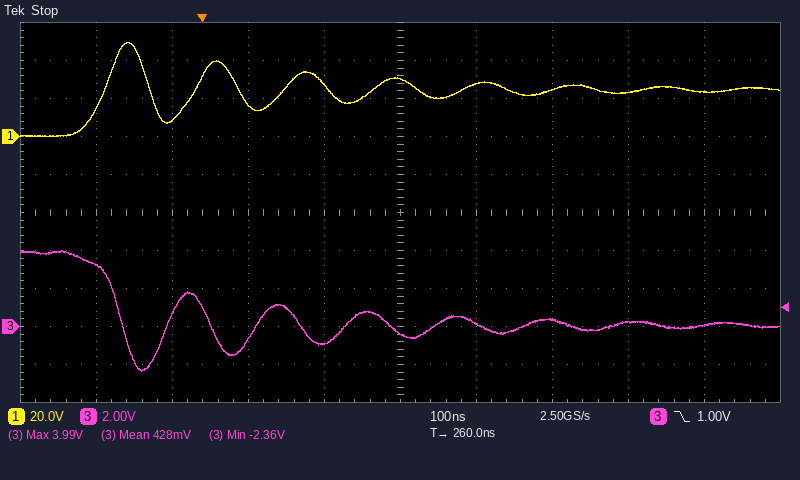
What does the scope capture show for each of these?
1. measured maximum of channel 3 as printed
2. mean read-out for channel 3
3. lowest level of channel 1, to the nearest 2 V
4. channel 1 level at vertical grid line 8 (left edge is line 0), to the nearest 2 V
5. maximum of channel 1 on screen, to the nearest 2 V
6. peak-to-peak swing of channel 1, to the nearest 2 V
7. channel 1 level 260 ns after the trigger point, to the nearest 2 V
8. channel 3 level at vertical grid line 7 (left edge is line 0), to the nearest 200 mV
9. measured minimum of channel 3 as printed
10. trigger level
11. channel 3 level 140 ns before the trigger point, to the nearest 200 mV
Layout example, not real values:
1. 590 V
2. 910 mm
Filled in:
1. 3.99 V
2. 428 mV
3. 0 V
4. 24 V
5. 50 V
6. 50 V
7. 30 V
8. 400 mV
9. -2.36 V
10. 1.00 V
11. 3.2 V
